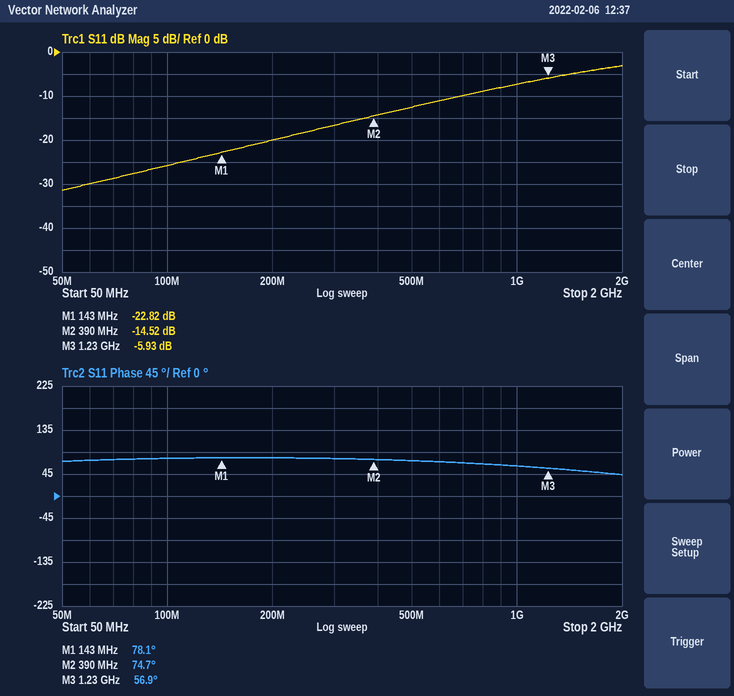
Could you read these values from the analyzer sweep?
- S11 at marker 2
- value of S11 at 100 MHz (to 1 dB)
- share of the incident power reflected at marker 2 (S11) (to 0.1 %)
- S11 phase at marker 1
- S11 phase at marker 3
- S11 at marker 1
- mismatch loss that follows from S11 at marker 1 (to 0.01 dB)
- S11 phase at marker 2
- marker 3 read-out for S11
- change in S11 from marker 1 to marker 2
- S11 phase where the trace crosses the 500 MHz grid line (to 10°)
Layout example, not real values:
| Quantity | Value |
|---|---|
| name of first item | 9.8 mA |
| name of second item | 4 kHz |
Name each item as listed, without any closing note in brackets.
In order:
| Quantity | Value |
|---|---|
| S11 at marker 2 | -14.52 dB |
| value of S11 at 100 MHz | -26 dB |
| share of the incident power reflected at marker 2 (S11) | 3.5 % |
| S11 phase at marker 1 | 78.1° |
| S11 phase at marker 3 | 56.9° |
| S11 at marker 1 | -22.82 dB |
| mismatch loss that follows from S11 at marker 1 | 0.02 dB |
| S11 phase at marker 2 | 74.7° |
| marker 3 read-out for S11 | -5.93 dB |
| change in S11 from marker 1 to marker 2 | 8.30 dB |
| S11 phase where the trace crosses the 500 MHz grid line | 70° |
